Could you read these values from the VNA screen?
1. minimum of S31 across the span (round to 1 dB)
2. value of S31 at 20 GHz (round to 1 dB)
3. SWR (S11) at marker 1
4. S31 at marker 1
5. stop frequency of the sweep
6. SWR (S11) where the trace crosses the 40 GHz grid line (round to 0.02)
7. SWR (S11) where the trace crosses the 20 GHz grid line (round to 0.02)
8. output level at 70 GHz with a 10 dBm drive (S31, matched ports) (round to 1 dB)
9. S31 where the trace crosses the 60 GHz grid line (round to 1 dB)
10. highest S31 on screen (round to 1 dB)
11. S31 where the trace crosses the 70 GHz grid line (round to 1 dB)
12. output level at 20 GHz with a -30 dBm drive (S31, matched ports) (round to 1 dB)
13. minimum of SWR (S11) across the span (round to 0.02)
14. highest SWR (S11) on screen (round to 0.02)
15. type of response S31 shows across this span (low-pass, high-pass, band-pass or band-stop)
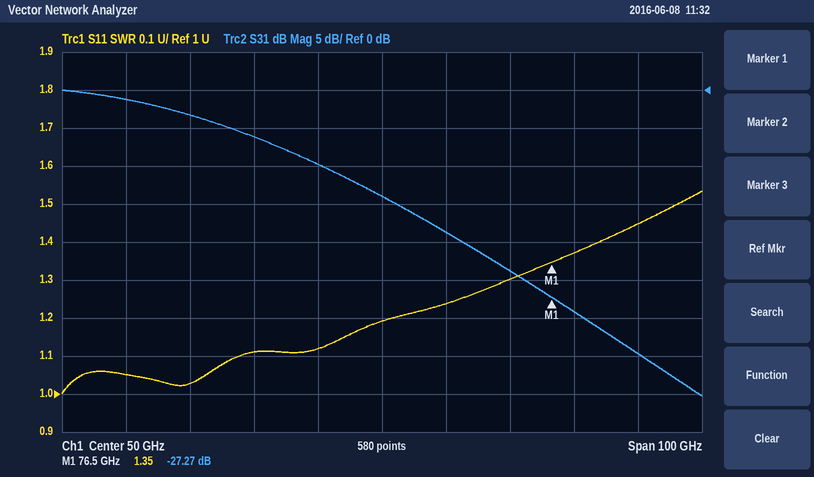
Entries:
-40 dB
-3 dB
1.35
-27.27 dB
100 GHz
1.12
1.02
-14 dBm
-19 dB
0 dB
-24 dB
-33 dBm
1.00
1.54
low-pass
